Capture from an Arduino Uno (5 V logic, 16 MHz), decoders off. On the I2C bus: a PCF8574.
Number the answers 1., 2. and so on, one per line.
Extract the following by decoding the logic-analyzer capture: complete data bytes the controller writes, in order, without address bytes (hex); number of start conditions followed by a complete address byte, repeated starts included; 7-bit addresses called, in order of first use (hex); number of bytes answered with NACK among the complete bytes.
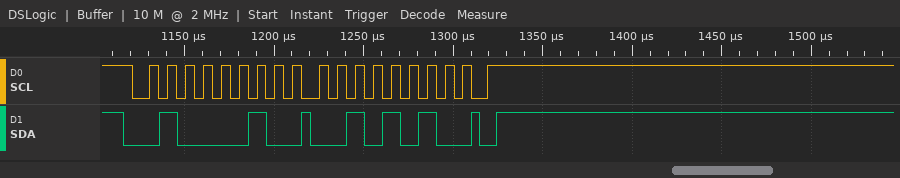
1. 2A
2. 1
3. 0x21
4. 0
